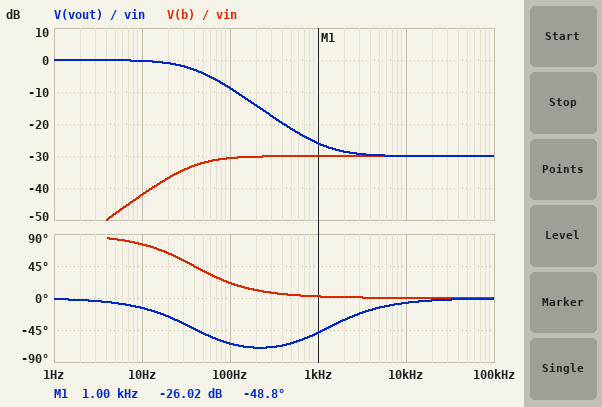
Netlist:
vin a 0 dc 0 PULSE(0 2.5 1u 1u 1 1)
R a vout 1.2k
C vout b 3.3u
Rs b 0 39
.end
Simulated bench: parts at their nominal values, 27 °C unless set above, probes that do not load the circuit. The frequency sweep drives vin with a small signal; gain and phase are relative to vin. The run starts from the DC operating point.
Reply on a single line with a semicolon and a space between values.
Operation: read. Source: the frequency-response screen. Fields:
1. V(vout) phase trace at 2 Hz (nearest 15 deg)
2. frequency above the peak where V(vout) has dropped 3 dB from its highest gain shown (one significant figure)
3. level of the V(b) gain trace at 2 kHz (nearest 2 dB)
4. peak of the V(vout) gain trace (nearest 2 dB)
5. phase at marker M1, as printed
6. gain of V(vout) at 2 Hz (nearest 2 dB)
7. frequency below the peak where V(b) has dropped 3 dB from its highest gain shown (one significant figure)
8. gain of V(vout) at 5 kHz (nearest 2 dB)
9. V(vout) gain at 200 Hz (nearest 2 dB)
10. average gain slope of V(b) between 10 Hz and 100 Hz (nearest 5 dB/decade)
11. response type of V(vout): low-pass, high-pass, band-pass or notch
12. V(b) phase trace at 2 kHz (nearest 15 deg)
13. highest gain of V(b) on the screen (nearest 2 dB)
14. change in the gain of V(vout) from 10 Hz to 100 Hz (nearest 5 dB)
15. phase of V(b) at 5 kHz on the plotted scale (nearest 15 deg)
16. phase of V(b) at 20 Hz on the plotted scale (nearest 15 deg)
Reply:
0 deg; 40 Hz; -30 dB; 0 dB; -48.8 deg; 0 dB; 40 Hz; -30 dB; -14 dB; 10 dB/decade; low-pass; 0 deg; -30 dB; -10 dB; 0 deg; 60 deg
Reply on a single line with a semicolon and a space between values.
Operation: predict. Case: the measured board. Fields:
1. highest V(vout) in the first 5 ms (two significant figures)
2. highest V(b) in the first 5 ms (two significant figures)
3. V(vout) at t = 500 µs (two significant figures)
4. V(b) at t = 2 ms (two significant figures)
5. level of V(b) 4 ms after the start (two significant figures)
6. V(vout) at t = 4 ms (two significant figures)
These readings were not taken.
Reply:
1.8 V; 79 mV; 360 mV; 48 mV; 30 mV; 1.6 V
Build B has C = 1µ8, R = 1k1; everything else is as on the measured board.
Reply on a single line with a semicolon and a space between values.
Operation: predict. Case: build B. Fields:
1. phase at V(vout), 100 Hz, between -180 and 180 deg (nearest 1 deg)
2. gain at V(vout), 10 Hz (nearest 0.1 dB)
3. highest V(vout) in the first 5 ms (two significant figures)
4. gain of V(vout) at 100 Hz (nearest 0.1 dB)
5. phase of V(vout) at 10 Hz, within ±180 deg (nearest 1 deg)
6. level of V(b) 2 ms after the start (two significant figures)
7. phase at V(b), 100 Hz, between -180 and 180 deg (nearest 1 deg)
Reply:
-50 deg; -0.1 dB; 2.3 V; -4.2 dB; -7 deg; 32 mV; 38 deg
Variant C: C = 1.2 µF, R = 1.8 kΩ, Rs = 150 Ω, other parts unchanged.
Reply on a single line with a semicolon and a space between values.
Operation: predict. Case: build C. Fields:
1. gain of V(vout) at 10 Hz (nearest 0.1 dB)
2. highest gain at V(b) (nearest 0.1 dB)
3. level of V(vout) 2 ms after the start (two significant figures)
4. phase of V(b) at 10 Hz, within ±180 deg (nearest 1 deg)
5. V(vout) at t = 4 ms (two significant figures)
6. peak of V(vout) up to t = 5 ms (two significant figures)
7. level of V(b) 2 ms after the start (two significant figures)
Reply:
-0.1 dB; -22.3 dB; 1.5 V; 82 deg; 2.1 V; 2.2 V; 82 mV
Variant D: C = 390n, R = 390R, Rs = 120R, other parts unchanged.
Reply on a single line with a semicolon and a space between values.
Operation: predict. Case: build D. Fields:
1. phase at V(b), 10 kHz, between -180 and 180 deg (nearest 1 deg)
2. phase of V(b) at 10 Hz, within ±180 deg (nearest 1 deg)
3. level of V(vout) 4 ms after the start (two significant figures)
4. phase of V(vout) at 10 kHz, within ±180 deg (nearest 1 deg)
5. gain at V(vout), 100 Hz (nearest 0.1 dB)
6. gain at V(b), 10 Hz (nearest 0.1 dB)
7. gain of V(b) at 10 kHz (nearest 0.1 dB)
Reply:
5 deg; 89 deg; 2.5 V; -14 deg; -0.1 dB; -50.6 dB; -12.6 dB
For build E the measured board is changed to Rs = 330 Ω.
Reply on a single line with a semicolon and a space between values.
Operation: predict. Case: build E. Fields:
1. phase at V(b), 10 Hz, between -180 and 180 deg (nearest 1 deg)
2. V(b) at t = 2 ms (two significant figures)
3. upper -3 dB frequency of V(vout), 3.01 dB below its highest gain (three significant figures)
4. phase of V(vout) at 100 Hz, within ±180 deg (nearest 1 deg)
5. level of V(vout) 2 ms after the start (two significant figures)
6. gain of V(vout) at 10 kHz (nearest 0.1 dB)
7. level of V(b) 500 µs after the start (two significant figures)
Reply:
72 deg; 360 mV; 33.1 Hz; -38 deg; 1.2 V; -13.3 dB; 490 mV
